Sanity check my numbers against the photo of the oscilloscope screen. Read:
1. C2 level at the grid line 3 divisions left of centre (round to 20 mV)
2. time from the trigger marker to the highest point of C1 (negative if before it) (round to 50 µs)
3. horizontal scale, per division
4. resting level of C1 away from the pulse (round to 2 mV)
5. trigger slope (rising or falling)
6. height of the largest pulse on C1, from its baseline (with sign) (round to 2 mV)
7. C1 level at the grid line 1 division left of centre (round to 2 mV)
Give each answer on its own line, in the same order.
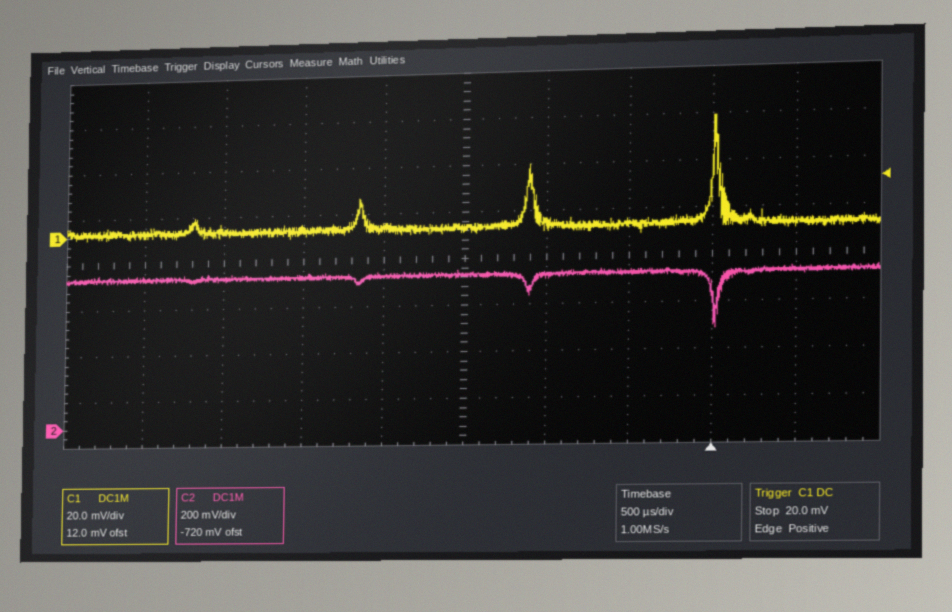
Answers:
640 mV
0 µs
500 µs
2 mV
rising
+46 mV
2 mV
